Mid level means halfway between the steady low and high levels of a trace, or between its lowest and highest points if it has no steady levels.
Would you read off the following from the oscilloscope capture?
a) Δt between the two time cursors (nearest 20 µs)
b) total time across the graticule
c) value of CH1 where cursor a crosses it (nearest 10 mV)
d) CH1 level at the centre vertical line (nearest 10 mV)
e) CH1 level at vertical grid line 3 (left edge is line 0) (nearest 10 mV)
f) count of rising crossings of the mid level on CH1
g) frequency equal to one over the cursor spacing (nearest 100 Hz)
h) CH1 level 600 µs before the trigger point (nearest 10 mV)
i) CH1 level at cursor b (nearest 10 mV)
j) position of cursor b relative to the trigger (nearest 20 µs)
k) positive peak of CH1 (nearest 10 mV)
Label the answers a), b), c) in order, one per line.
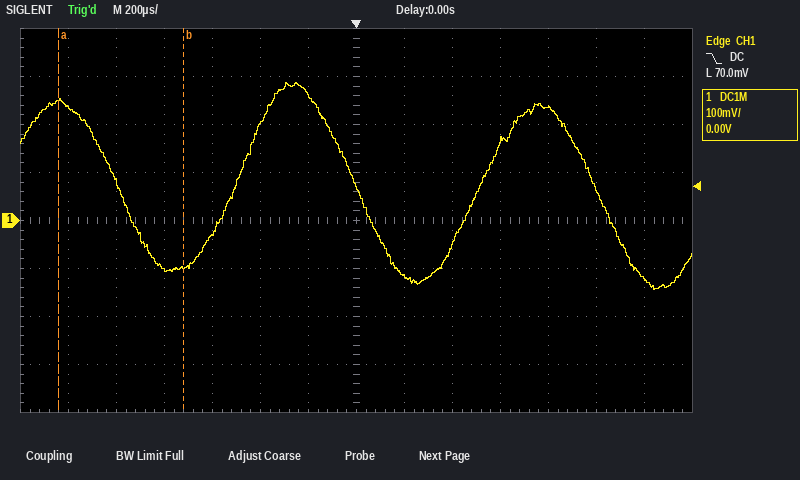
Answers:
a) 520 µs
b) 2.8 ms
c) 250 mV
d) 70 mV
e) -100 mV
f) 2
g) 1.9 kHz
h) -30 mV
i) -100 mV
j) -720 µs
k) 290 mV
